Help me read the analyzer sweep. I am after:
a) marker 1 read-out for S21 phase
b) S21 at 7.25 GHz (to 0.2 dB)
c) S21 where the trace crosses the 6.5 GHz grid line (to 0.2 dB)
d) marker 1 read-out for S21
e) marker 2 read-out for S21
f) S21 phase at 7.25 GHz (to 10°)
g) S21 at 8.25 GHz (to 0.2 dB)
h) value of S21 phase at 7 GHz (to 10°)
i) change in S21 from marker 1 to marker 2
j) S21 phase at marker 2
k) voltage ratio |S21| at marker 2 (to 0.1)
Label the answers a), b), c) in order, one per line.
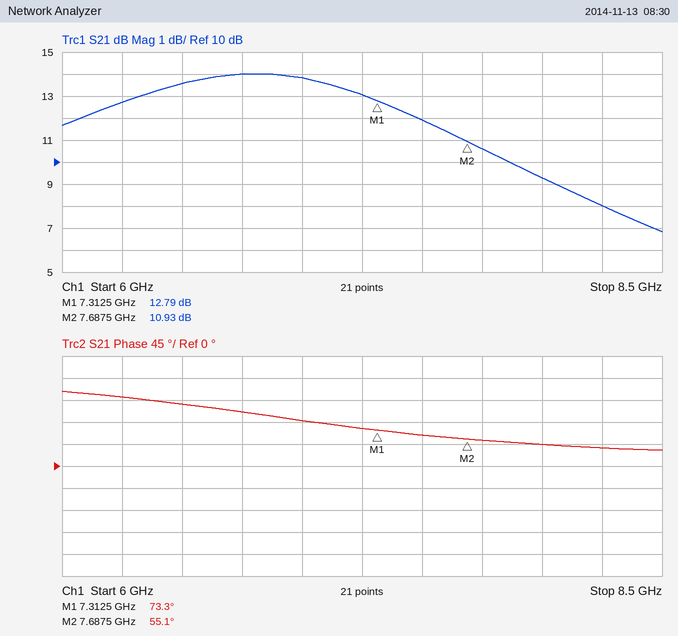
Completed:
a) 73.3°
b) 13.0 dB
c) 13.6 dB
d) 12.79 dB
e) 10.93 dB
f) 80°
g) 8.0 dB
h) 90°
i) -1.86 dB
j) 55.1°
k) 3.5
